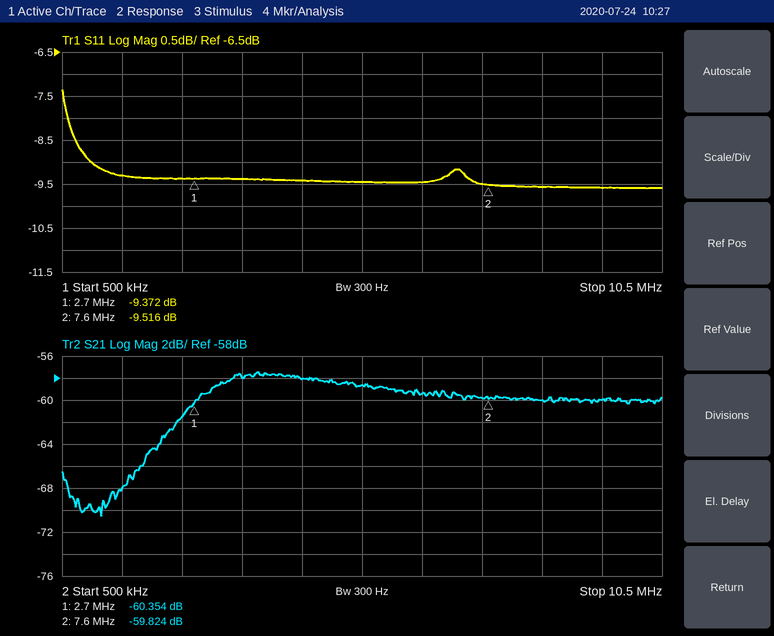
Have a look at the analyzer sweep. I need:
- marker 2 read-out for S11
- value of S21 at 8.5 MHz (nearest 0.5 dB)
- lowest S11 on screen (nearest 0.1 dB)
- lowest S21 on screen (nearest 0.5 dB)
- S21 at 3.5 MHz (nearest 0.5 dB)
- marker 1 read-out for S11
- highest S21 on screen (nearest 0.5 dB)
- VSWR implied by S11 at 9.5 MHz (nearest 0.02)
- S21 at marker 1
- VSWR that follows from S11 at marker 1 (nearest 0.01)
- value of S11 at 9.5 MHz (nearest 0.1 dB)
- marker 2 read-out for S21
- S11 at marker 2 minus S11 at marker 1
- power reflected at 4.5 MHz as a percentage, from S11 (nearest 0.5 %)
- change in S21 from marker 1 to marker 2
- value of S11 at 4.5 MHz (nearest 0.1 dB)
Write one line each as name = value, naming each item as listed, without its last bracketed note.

marker 2 read-out for S11 = -9.516 dB
value of S21 at 8.5 MHz = -60.0 dB
lowest S11 on screen = -9.6 dB
lowest S21 on screen = -70.5 dB
S21 at 3.5 MHz = -58.0 dB
marker 1 read-out for S11 = -9.372 dB
highest S21 on screen = -57.5 dB
VSWR implied by S11 at 9.5 MHz = 2.00
S21 at marker 1 = -60.354 dB
VSWR that follows from S11 at marker 1 = 2.03
value of S11 at 9.5 MHz = -9.6 dB
marker 2 read-out for S21 = -59.824 dB
S11 at marker 2 minus S11 at marker 1 = -0.144 dB
power reflected at 4.5 MHz as a percentage, from S11 = 11.5 %
change in S21 from marker 1 to marker 2 = 0.530 dB
value of S11 at 4.5 MHz = -9.4 dB
